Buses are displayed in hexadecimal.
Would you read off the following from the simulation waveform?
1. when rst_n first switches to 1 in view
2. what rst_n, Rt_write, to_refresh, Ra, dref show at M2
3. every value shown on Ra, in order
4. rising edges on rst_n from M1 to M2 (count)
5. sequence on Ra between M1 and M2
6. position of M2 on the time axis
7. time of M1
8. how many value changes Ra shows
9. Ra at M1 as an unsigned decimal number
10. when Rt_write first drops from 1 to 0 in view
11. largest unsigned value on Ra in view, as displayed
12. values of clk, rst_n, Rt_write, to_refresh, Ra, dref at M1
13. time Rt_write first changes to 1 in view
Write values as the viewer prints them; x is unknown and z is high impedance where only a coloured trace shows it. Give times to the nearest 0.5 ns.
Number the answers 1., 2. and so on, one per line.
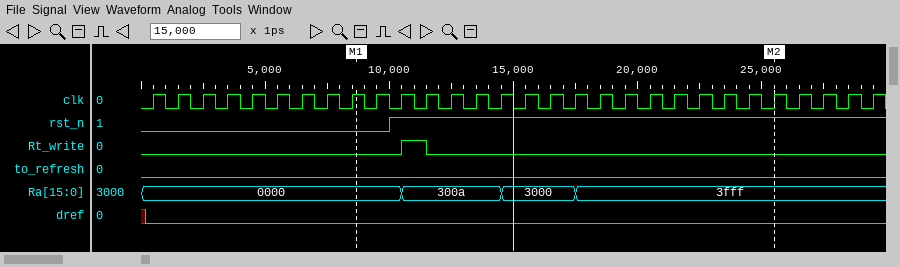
1. 10 ns
2. rst_n=1, Rt_write=0, to_refresh=0, Ra=3fff, dref=0
3. 0000, 300a, 3000, 3fff
4. 1
5. 0000, 300a, 3000, 3fff
6. 25.5 ns
7. 8.5 ns
8. 3
9. 0
10. 11.5 ns
11. 3fff
12. clk=1, rst_n=0, Rt_write=0, to_refresh=0, Ra=0000, dref=0
13. 10.5 ns
